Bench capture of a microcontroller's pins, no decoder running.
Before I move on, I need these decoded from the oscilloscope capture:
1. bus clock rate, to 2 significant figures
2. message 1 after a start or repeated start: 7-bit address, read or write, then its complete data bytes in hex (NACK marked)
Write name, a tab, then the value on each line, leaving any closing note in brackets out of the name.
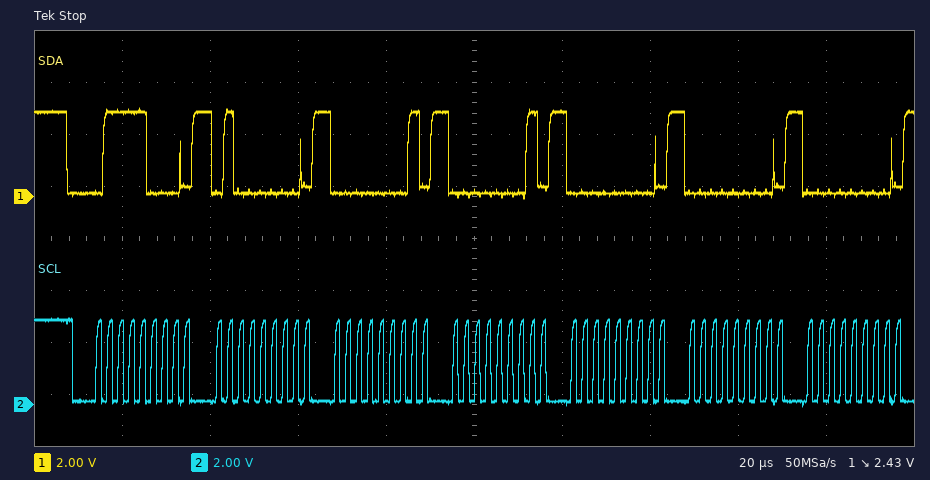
bus clock rate, to 2 significant figures	400 kHz
message 1 after a start or repeated start: 7-bit address, read or write, then its complete data bytes in hex	0x3C write: 40 01 01 00 00 00
